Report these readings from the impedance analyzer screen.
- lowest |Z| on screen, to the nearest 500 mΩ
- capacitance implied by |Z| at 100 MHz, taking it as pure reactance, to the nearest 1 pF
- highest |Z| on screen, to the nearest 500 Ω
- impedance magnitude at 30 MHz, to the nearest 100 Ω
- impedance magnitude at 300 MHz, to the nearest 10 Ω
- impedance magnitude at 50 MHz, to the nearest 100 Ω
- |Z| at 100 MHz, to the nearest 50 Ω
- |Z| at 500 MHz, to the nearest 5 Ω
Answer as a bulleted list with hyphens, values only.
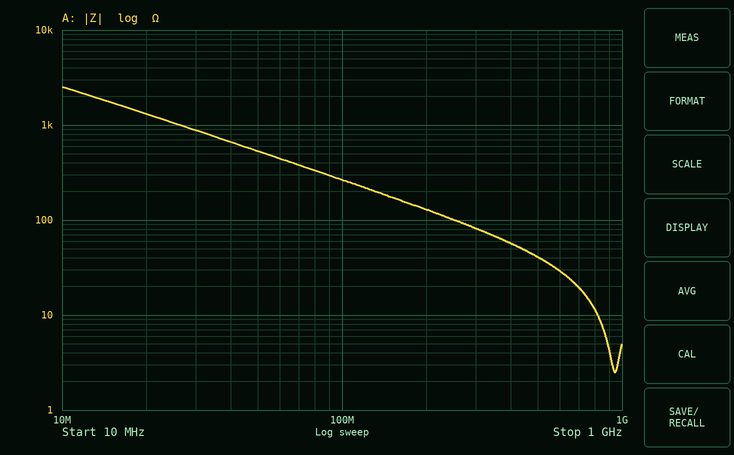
- 2.5 Ω
- 6 pF
- 2.5 kΩ
- 900 Ω
- 80 Ω
- 500 Ω
- 250 Ω
- 40 Ω
